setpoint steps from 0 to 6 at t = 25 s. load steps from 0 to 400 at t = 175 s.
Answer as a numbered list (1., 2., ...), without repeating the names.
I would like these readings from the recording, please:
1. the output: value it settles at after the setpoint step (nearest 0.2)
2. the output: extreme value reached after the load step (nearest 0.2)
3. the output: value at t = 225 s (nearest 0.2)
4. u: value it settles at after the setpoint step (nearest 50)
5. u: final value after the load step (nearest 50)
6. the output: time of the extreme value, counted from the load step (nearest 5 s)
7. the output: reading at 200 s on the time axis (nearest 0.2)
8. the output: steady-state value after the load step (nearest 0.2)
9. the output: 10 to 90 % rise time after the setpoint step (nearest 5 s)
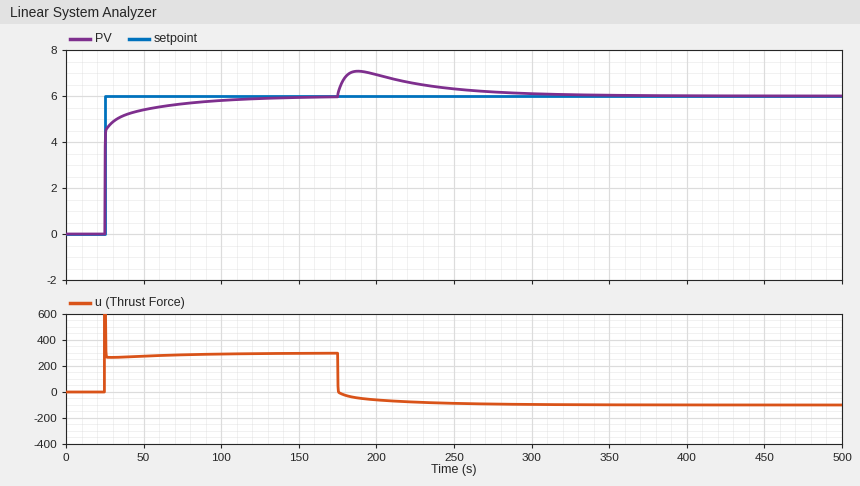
1. 6.0
2. 7.0
3. 6.6
4. 300
5. -100
6. 15 s
7. 7.0
8. 6.0
9. 25 s
